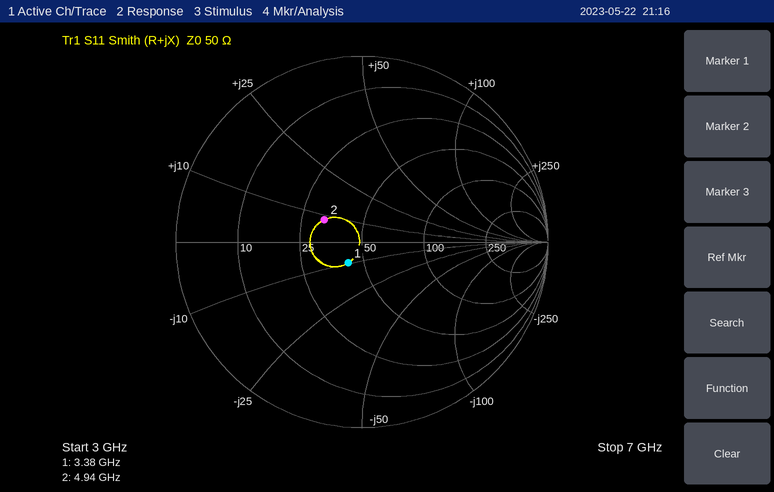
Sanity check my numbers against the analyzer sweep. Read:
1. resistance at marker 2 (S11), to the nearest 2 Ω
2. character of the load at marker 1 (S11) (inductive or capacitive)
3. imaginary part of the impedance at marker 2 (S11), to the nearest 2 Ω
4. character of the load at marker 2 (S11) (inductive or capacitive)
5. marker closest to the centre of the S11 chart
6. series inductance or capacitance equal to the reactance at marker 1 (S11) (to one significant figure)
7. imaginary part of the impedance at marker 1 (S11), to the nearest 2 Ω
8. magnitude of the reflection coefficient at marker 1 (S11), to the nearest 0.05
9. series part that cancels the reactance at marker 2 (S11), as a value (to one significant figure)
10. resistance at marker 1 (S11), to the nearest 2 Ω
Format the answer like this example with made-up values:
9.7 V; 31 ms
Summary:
32 Ω; capacitive; +8 Ω; inductive; marker 1; 5 pF; -10 Ω; 0.15; 4 pF; 42 Ω
